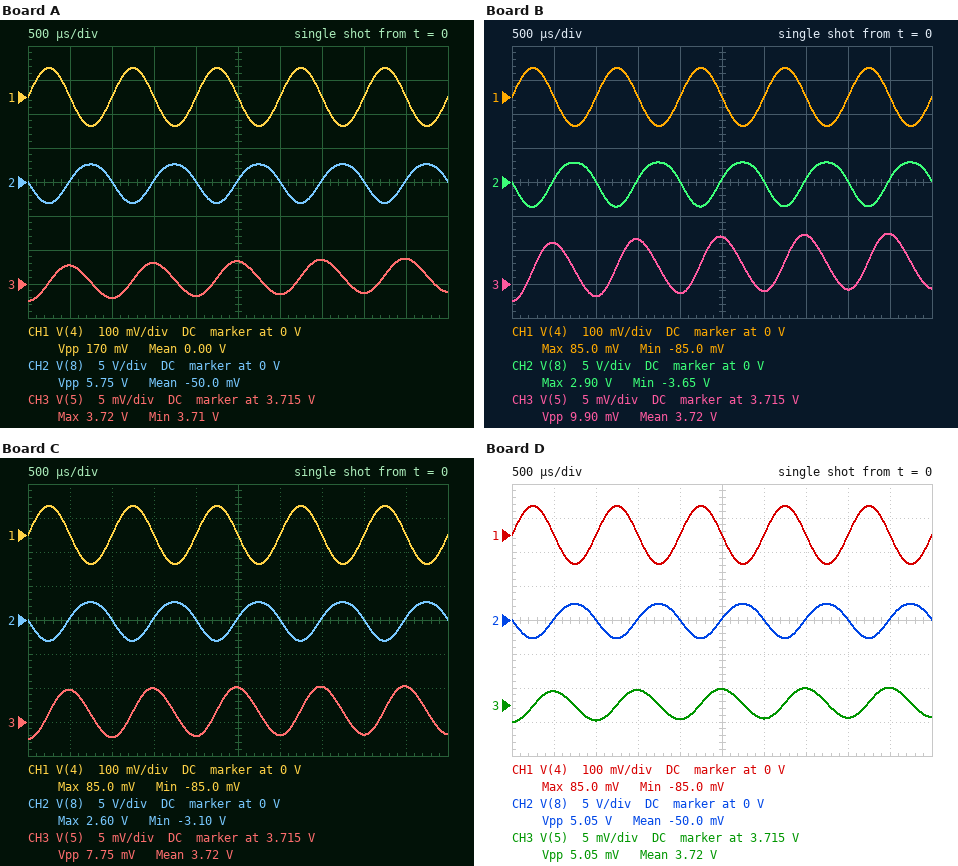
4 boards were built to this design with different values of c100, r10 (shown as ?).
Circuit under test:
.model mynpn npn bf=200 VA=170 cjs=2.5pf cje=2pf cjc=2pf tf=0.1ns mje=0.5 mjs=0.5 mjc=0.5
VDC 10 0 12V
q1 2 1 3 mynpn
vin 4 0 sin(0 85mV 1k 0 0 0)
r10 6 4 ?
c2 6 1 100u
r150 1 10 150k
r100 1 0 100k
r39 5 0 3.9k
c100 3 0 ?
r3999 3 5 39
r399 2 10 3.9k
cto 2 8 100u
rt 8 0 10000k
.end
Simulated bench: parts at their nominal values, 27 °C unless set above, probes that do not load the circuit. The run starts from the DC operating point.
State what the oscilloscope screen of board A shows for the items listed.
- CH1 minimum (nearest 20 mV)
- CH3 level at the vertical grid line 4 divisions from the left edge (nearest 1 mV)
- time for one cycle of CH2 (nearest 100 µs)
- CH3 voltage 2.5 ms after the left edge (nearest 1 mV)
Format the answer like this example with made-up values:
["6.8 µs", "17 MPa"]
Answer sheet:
["-80 mV", "3.713 V", "1.0 ms", "3.718 V"]
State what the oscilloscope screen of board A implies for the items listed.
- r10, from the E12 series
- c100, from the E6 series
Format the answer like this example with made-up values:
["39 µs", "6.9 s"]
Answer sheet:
["15 kΩ", "47 µF"]
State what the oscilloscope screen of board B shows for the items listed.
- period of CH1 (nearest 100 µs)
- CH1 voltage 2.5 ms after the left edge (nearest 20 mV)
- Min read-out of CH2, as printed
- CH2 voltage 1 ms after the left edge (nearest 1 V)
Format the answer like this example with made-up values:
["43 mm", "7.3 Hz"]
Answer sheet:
["1.0 ms", "0 V", "-3.65 V", "0 V"]
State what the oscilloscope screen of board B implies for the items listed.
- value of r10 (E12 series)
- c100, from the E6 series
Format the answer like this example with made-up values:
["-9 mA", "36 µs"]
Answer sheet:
["12 kΩ", "33 µF"]
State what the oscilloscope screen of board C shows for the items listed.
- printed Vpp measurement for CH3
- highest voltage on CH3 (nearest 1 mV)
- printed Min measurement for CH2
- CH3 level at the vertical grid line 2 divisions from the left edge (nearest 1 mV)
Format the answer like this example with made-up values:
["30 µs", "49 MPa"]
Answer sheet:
["7.75 mV", "3.720 V", "-3.10 V", "3.713 V"]
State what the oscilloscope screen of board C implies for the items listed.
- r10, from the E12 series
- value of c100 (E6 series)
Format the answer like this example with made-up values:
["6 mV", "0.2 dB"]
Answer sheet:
["15 kΩ", "33 µF"]
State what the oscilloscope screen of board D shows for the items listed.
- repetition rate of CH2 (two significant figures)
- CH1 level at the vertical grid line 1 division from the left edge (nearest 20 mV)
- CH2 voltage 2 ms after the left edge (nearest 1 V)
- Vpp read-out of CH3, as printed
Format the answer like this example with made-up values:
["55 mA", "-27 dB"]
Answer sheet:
["1.0 kHz", "0 V", "0 V", "5.05 mV"]
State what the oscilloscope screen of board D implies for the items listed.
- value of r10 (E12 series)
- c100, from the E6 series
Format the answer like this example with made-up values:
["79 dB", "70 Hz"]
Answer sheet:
["18 kΩ", "47 µF"]
